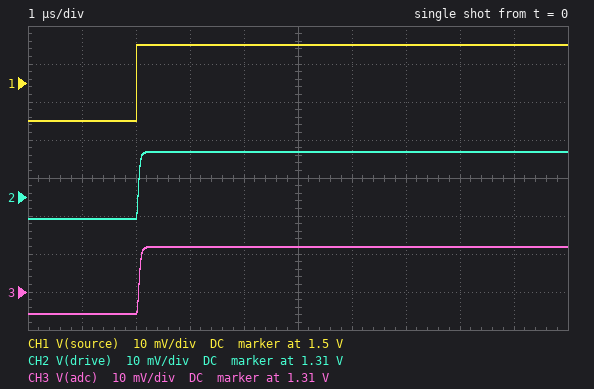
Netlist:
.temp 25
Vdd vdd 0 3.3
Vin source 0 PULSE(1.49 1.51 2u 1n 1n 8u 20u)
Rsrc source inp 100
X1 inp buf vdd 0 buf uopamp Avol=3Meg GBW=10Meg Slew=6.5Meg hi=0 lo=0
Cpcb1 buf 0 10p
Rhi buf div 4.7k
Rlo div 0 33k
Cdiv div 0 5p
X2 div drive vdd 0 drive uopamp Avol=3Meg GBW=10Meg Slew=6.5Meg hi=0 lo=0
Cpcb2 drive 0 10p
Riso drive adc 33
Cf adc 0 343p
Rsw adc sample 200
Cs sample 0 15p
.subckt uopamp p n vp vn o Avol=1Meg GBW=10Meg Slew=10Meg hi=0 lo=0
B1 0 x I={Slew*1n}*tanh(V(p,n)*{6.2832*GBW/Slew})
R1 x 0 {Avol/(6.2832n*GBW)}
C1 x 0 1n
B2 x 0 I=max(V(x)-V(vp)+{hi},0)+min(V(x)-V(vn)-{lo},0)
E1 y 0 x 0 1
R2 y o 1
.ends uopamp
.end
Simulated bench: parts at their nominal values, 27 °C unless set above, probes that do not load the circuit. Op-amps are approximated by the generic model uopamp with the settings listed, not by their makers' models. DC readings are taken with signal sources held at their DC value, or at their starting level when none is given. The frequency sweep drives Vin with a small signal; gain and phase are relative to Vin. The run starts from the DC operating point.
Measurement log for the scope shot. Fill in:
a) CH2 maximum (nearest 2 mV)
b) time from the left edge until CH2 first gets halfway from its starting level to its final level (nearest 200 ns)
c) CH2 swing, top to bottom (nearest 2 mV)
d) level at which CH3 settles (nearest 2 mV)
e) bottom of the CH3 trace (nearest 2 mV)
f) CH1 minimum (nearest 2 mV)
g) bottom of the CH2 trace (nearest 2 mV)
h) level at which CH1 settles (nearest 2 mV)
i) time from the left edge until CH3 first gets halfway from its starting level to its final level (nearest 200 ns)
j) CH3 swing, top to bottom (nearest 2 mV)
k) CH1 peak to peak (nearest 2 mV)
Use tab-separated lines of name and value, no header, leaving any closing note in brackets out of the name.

CH2 maximum	1.322 V
time from the left edge until CH2 first gets halfway from its starting level to its final level	2.0 µs
CH2 swing, top to bottom	18 mV
level at which CH3 settles	1.322 V
bottom of the CH3 trace	1.304 V
CH1 minimum	1.490 V
bottom of the CH2 trace	1.304 V
level at which CH1 settles	1.510 V
time from the left edge until CH3 first gets halfway from its starting level to its final level	2.0 µs
CH3 swing, top to bottom	18 mV
CH1 peak to peak	20 mV
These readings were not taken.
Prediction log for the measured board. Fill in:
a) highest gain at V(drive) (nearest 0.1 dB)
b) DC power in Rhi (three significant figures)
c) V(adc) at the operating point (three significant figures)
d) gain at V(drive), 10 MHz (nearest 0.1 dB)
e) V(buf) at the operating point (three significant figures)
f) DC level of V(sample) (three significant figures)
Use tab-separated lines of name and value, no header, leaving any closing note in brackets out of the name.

highest gain at V(drive)	-1.2 dB
DC power in Rhi	7.34 µW
V(adc) at the operating point	1.30 V
gain at V(drive), 10 MHz	-11.4 dB
V(buf) at the operating point	1.49 V
DC level of V(sample)	1.30 V
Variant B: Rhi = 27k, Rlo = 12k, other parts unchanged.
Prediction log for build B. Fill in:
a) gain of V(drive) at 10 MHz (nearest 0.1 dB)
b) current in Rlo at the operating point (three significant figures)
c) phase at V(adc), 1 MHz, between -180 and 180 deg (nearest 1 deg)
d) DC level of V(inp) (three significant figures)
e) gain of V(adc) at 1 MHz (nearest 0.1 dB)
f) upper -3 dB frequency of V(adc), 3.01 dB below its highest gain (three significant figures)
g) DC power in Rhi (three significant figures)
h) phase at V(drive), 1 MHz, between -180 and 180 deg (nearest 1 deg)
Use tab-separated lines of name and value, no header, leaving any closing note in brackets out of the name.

gain of V(drive) at 10 MHz	-25.2 dB
current in Rlo at the operating point	38.2 µA
phase at V(adc), 1 MHz, between -180 and 180 deg	-30 deg
DC level of V(inp)	1.49 V
gain of V(adc) at 1 MHz	-10.6 dB
upper -3 dB frequency of V(adc), 3.01 dB below its highest gain	2.99 MHz
DC power in Rhi	39.4 µW
phase at V(drive), 1 MHz, between -180 and 180 deg	-26 deg
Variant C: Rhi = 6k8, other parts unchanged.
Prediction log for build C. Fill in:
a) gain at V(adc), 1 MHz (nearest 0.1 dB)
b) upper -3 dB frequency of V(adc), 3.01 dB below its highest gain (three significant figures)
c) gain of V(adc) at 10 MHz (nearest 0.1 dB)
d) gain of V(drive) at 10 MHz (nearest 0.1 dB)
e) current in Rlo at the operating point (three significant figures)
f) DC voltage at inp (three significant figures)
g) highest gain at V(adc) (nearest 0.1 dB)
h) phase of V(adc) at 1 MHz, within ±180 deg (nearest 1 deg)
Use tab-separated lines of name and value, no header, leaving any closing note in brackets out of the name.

gain at V(adc), 1 MHz	-1.9 dB
upper -3 dB frequency of V(adc), 3.01 dB below its highest gain	3.73 MHz
gain of V(adc) at 10 MHz	-15.7 dB
gain of V(drive) at 10 MHz	-13.8 dB
current in Rlo at the operating point	37.4 µA
DC voltage at inp	1.49 V
highest gain at V(adc)	-1.6 dB
phase of V(adc) at 1 MHz, within ±180 deg	-26 deg
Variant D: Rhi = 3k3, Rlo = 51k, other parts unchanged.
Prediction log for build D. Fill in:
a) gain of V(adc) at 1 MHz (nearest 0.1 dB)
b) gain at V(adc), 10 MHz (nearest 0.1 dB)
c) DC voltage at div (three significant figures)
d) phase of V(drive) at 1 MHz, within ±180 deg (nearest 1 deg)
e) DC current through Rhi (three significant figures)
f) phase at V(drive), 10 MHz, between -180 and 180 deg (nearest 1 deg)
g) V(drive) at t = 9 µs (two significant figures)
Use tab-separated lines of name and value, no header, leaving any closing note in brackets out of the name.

gain of V(adc) at 1 MHz	-0.7 dB
gain at V(adc), 10 MHz	-11.4 dB
DC voltage at div	1.40 V
phase of V(drive) at 1 MHz, within ±180 deg	-17 deg
DC current through Rhi	27.4 µA
phase at V(drive), 10 MHz, between -180 and 180 deg	-135 deg
V(drive) at t = 9 µs	1.4 V
